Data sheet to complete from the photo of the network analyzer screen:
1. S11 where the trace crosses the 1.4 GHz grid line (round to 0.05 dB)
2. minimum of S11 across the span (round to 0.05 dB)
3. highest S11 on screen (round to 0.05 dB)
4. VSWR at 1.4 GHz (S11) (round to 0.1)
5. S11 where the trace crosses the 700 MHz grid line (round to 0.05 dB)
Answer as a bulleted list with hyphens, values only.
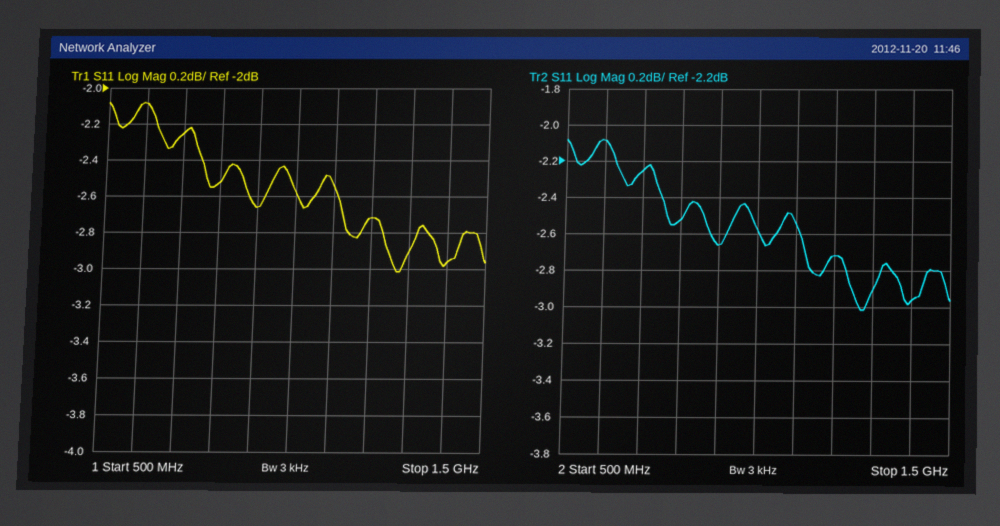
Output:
- -2.95 dB
- -3.00 dB
- -2.10 dB
- 5.9
- -2.25 dB
